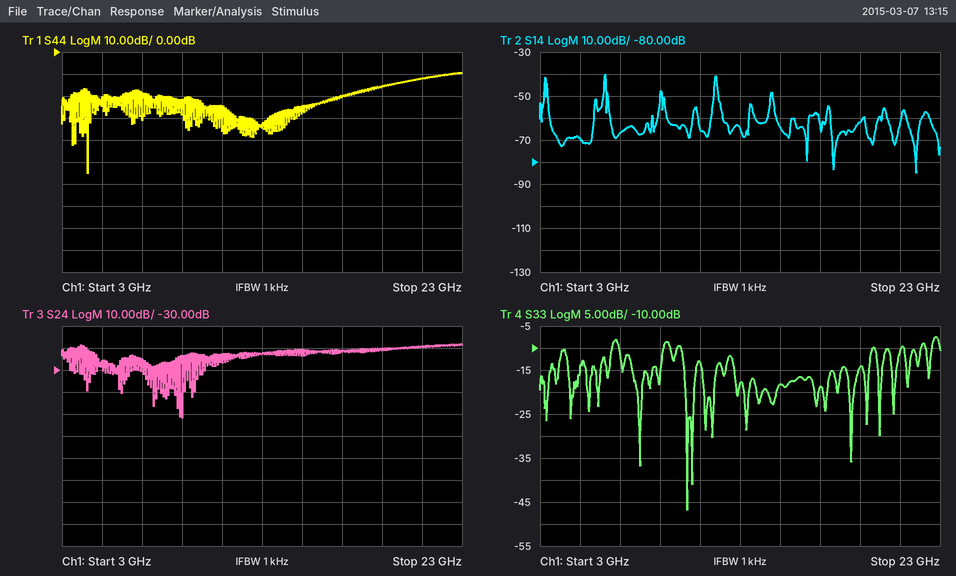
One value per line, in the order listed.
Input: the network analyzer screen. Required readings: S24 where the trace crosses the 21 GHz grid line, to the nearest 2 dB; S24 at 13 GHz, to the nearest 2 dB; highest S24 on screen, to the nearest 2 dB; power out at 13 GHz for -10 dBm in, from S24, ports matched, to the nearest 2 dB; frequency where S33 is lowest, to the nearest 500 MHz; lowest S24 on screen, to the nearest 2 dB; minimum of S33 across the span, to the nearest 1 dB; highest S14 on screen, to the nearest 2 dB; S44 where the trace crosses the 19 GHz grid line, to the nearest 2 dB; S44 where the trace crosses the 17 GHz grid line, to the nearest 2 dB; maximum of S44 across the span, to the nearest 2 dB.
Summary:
-20 dB
-22 dB
-18 dB
-32 dBm
10.5 GHz
-52 dB
-47 dB
-40 dB
-16 dB
-20 dB
-10 dB
